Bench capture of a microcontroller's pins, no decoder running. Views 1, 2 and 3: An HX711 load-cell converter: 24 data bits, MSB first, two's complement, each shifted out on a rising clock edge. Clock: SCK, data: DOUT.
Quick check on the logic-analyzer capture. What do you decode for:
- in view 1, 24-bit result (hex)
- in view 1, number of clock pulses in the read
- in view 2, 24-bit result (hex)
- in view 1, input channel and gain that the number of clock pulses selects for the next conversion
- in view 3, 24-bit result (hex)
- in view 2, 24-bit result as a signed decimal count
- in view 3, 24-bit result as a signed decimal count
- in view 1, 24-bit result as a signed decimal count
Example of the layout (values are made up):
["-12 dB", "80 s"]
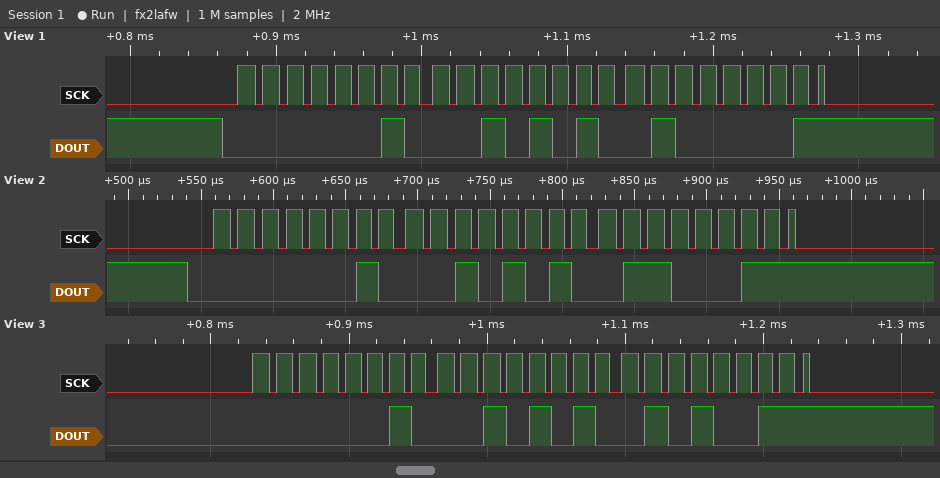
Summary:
["0x022A41", "25", "0x022A63", "channel A, gain 128", "0x022A53", "141923", "141907", "141889"]
